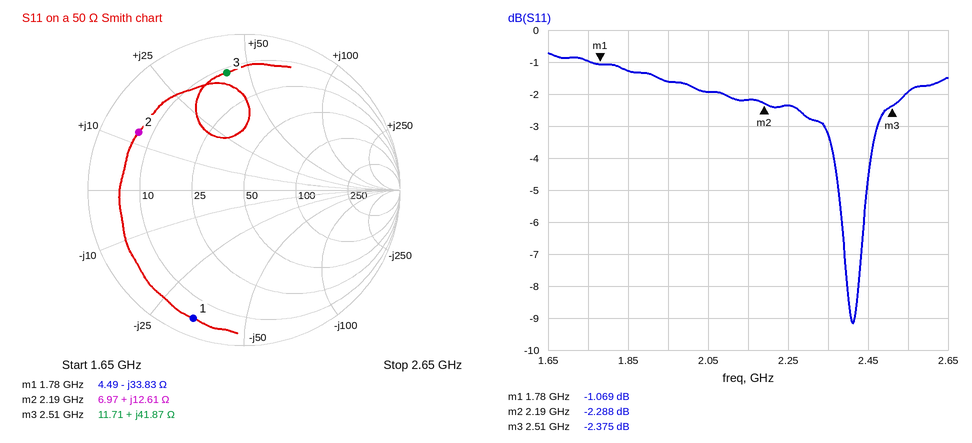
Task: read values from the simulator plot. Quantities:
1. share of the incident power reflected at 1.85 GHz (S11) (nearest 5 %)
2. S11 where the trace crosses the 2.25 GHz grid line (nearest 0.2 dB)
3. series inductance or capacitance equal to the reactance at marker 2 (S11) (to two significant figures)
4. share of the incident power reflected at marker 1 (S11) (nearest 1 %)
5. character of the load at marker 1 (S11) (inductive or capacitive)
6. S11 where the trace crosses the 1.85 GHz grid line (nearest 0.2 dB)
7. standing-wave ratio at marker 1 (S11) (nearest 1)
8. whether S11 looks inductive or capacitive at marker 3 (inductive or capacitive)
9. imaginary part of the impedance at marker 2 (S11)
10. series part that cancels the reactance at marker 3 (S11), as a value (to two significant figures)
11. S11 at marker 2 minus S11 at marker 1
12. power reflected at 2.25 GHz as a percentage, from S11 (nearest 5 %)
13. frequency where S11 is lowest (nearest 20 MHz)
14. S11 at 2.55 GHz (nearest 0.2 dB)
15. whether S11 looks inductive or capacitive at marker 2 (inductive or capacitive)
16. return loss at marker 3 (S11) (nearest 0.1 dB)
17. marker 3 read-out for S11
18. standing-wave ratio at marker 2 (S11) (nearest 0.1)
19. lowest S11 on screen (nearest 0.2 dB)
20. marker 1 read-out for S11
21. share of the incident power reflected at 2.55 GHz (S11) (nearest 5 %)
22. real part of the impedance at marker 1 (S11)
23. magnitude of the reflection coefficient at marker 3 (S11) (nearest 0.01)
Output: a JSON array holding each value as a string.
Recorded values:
["75 %", "-2.4 dB", "920 pH", "78 %", "capacitive", "-1.2 dB", "16", "inductive", "+12.61 Ω", "1.5 pF", "-1.219 dB", "60 %", "2.42 GHz", "-2.0 dB", "inductive", "2.4 dB", "-2.375 dB", "7.6", "-9.2 dB", "-1.069 dB", "65 %", "4.49 Ω", "0.76"]
